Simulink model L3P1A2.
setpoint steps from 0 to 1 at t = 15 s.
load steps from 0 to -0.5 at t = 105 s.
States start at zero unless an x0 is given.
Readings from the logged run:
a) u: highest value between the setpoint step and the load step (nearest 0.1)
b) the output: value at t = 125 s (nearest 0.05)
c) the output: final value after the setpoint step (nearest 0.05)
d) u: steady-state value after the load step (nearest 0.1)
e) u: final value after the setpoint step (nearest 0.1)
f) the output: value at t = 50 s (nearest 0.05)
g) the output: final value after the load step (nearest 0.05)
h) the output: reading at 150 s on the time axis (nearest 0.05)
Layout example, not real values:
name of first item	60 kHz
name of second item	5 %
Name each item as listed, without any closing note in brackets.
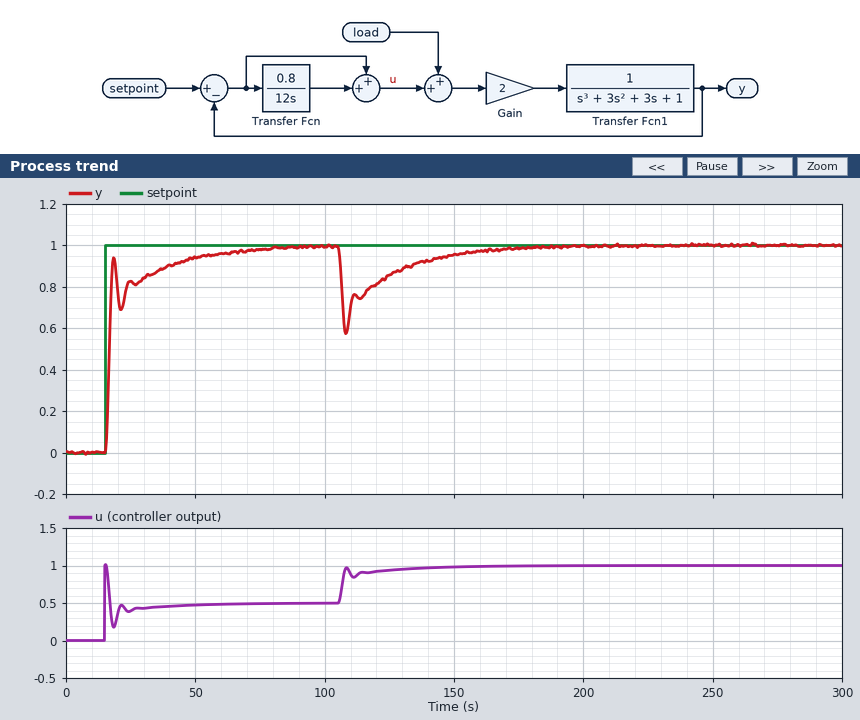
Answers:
u: highest value between the setpoint step and the load step	1.0
the output: value at t = 125 s	0.85
the output: final value after the setpoint step	1.00
u: steady-state value after the load step	1.0
u: final value after the setpoint step	0.5
the output: value at t = 50 s	0.95
the output: final value after the load step	1.00
the output: reading at 150 s on the time axis	0.95
